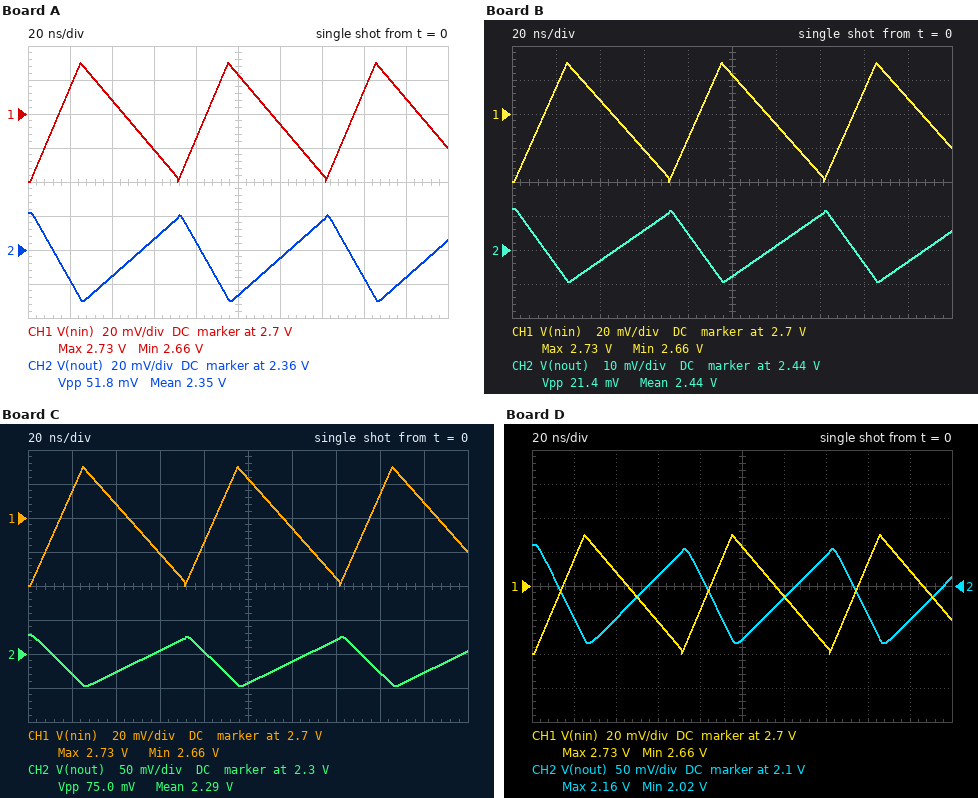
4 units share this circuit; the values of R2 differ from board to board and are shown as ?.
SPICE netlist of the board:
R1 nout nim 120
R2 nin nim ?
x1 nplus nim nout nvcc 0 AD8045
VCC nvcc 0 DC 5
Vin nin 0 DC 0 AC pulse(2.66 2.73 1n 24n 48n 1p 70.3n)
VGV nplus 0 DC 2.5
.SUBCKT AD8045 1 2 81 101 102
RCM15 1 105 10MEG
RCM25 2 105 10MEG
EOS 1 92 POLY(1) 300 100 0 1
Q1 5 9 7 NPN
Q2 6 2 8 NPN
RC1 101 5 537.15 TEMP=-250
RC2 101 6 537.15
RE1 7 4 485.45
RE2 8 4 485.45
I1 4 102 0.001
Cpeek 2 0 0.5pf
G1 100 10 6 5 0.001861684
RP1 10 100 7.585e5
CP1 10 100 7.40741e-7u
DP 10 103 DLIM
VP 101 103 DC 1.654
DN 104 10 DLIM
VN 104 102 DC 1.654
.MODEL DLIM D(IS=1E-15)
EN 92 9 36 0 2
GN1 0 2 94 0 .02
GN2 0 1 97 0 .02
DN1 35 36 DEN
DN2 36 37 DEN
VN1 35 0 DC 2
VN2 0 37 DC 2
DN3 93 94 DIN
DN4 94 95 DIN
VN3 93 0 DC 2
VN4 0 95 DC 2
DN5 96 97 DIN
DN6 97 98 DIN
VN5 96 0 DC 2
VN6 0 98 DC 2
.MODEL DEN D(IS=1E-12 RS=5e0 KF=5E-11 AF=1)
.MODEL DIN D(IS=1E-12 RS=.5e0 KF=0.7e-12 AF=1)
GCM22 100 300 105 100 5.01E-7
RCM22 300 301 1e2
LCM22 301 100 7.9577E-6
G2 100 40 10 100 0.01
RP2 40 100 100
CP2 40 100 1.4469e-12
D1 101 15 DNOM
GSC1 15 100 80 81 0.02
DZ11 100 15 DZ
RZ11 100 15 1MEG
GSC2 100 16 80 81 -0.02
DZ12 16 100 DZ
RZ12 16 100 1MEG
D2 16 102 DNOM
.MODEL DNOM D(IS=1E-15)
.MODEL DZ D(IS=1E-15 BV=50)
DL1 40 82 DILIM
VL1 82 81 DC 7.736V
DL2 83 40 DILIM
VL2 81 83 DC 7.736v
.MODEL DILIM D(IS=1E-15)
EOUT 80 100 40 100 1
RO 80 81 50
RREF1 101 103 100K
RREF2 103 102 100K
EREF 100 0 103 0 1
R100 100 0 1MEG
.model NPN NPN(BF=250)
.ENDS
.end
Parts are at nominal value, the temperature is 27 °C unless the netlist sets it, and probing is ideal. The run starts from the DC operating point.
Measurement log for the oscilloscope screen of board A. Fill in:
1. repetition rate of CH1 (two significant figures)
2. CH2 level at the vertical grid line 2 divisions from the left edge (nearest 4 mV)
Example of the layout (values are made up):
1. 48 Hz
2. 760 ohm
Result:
1. 14 MHz
2. 2.344 V
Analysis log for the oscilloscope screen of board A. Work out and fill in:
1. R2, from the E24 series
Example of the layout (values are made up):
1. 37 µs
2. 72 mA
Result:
1. 160 Ω
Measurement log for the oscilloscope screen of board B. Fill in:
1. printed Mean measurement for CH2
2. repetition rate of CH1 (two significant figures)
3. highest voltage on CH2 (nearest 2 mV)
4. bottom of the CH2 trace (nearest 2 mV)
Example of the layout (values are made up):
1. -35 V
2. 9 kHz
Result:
1. 2.44 V
2. 14 MHz
3. 2.452 V
4. 2.430 V
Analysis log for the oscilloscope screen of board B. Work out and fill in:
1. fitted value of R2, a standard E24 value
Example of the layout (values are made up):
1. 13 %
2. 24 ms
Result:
1. 390 Ω
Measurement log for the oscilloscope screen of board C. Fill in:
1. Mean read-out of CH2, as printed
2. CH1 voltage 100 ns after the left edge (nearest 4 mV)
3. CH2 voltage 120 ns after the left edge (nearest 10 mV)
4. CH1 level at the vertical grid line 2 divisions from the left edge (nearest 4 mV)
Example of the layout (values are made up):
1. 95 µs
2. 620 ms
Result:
1. 2.29 V
2. 2.724 V
3. 2.29 V
4. 2.708 V
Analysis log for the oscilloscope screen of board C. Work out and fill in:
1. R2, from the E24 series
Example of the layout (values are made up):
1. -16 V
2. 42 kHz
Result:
1. 110 Ω
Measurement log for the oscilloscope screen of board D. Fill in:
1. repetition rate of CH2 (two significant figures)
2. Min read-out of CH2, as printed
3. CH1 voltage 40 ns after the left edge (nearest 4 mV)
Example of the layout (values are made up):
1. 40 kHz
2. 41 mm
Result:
1. 14 MHz
2. 2.02 V
3. 2.708 V
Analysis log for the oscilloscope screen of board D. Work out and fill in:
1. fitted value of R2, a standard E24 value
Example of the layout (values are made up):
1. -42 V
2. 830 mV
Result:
1. 56 Ω
